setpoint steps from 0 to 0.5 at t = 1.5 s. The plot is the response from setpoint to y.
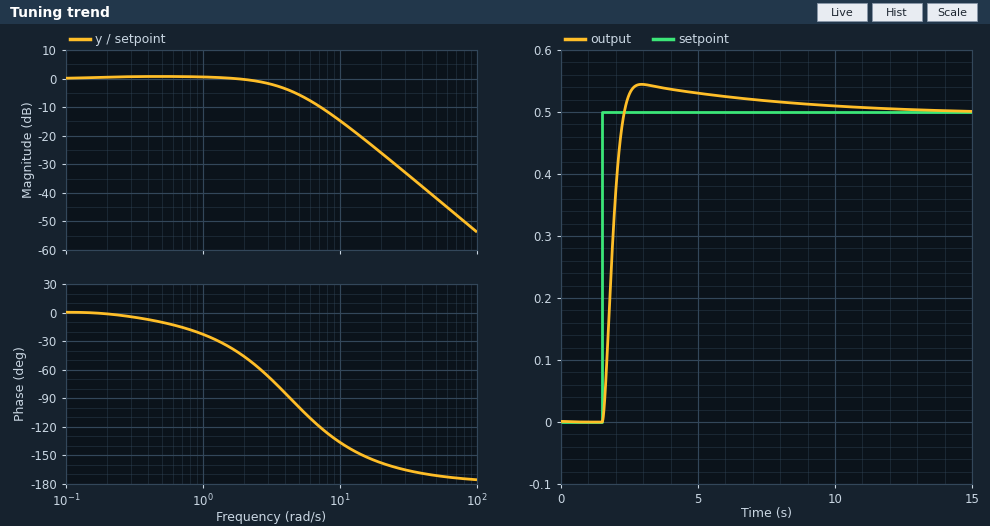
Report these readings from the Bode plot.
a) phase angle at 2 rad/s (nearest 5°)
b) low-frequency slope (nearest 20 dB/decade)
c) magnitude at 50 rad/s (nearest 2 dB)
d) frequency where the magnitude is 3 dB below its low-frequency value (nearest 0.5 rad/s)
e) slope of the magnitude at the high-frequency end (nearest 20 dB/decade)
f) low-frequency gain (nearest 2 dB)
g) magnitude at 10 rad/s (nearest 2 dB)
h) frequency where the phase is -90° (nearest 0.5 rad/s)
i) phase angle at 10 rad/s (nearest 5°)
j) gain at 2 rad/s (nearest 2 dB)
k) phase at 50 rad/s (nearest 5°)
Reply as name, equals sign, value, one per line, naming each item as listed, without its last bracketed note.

phase angle at 2 rad/s = -45°
low-frequency slope = 0 dB/decade
magnitude at 50 rad/s = -42 dB
frequency where the magnitude is 3 dB below its low-frequency value = 3.5 rad/s
slope of the magnitude at the high-frequency end = -40 dB/decade
low-frequency gain = 0 dB
magnitude at 10 rad/s = -14 dB
frequency where the phase is -90° = 4.5 rad/s
phase angle at 10 rad/s = -135°
gain at 2 rad/s = 0 dB
phase at 50 rad/s = -170°
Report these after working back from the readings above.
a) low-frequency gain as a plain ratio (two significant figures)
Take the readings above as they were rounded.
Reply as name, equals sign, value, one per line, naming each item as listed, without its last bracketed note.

low-frequency gain as a plain ratio = 1.0
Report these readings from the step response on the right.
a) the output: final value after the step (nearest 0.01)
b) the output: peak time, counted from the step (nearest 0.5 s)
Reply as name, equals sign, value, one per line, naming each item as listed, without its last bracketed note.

the output: final value after the step = 0.50
the output: peak time, counted from the step = 1.5 s
